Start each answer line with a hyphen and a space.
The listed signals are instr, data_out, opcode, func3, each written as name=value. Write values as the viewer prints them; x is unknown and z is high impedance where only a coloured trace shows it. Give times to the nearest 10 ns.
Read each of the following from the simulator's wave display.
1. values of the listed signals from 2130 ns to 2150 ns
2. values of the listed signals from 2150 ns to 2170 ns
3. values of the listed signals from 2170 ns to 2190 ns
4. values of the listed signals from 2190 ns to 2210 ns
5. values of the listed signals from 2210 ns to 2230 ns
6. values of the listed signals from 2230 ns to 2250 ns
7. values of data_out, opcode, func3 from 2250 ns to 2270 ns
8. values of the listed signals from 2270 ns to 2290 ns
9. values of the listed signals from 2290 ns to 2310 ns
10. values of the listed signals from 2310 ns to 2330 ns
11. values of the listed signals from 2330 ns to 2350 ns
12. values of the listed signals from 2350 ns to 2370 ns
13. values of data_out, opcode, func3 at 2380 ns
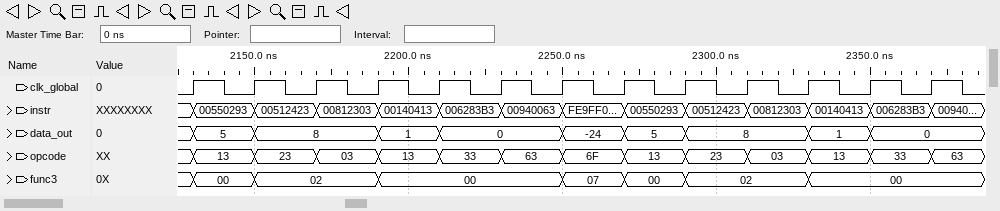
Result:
- instr=00550293, data_out=5, opcode=13, func3=00
- instr=00512423, data_out=8, opcode=23, func3=02
- instr=00812303, data_out=8, opcode=03, func3=02
- instr=00140413, data_out=1, opcode=13, func3=00
- instr=006283B3, data_out=0, opcode=33, func3=00
- instr=00940063, data_out=0, opcode=63, func3=00
- data_out=-24, opcode=6F, func3=07
- instr=00550293, data_out=5, opcode=13, func3=00
- instr=00512423, data_out=8, opcode=23, func3=02
- instr=00812303, data_out=8, opcode=03, func3=02
- instr=00140413, data_out=1, opcode=13, func3=00
- instr=006283B3, data_out=0, opcode=33, func3=00
- data_out=0, opcode=63, func3=00
